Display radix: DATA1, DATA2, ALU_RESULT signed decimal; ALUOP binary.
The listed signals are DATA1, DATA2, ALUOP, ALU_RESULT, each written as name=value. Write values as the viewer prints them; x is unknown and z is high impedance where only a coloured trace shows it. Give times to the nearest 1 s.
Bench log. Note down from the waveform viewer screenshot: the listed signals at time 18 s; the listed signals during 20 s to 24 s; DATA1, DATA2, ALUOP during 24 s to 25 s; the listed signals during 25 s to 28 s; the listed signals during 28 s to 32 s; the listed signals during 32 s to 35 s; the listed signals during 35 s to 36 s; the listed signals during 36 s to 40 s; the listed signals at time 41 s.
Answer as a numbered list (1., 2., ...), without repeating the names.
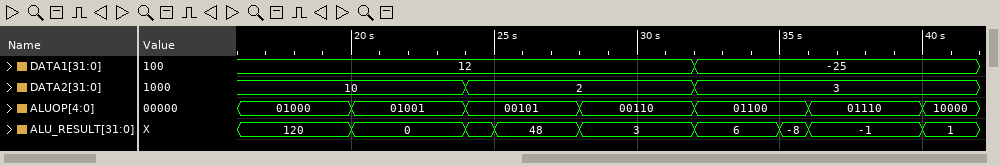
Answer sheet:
1. DATA1=12, DATA2=10, ALUOP=01000, ALU_RESULT=120
2. DATA1=12, DATA2=10, ALUOP=01001, ALU_RESULT=0
3. DATA1=12, DATA2=2, ALUOP=00101
4. DATA1=12, DATA2=2, ALUOP=00101, ALU_RESULT=48
5. DATA1=12, DATA2=2, ALUOP=00110, ALU_RESULT=3
6. DATA1=-25, DATA2=3, ALUOP=01100, ALU_RESULT=6
7. DATA1=-25, DATA2=3, ALUOP=01100, ALU_RESULT=-8
8. DATA1=-25, DATA2=3, ALUOP=01110, ALU_RESULT=-1
9. DATA1=-25, DATA2=3, ALUOP=10000, ALU_RESULT=1
